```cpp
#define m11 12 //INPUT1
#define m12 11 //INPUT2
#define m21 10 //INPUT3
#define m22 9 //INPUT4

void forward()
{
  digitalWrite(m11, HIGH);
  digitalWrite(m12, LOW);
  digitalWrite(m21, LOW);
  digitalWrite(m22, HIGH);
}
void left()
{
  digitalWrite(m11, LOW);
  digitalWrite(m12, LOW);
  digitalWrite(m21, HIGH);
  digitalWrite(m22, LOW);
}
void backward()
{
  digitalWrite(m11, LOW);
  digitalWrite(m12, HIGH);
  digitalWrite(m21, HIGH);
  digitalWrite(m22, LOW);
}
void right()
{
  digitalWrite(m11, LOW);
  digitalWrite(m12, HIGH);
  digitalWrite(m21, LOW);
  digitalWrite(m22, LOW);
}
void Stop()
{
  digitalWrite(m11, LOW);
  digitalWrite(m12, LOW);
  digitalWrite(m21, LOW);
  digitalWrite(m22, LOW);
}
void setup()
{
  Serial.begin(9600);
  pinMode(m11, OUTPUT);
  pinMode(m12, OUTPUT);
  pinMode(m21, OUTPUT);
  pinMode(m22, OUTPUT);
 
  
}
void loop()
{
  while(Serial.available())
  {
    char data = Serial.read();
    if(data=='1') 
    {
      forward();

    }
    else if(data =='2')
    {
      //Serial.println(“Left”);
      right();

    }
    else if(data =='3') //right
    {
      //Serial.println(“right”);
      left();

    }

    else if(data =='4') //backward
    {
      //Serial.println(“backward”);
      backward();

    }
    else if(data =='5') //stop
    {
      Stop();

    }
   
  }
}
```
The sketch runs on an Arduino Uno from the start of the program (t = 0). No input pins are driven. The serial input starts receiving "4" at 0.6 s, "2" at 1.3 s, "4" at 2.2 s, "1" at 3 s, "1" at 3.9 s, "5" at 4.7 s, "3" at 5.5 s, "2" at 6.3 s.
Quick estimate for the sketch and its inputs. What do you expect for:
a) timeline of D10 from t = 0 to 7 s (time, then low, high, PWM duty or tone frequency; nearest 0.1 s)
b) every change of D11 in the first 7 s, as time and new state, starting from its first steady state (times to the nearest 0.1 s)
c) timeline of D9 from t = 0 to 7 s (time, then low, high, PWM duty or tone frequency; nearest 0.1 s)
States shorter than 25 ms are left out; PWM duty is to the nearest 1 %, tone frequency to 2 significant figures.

0 s low; 0.6 s high; 1.3 s low; 2.2 s high; 3 s low; 5.5 s high; 6.3 s low
0 s low; 0.6 s high; 3 s low; 6.3 s high
0 s low; 3 s high; 4.7 s low
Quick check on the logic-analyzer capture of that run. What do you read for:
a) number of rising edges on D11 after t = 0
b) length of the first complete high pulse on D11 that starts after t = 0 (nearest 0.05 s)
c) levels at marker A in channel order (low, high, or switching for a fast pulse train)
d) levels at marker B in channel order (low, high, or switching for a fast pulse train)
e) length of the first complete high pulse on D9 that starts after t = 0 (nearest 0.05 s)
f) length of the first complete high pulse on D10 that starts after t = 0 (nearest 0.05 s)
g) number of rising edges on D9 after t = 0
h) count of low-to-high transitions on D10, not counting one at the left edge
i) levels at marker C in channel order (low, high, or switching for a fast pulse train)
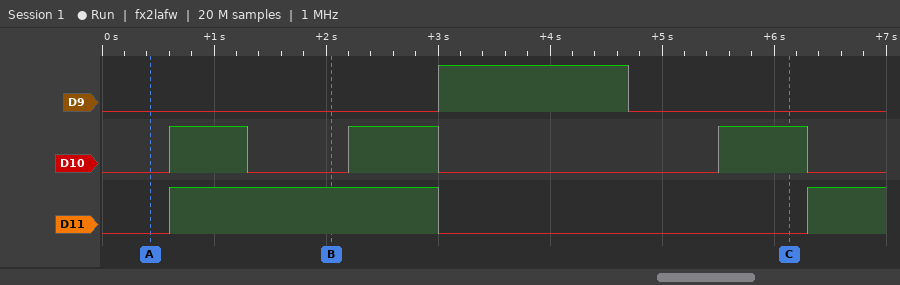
2
2.40 s
D9 low, D10 low, D11 low
D9 low, D10 low, D11 high
1.70 s
0.70 s
1
3
D9 low, D10 high, D11 low
